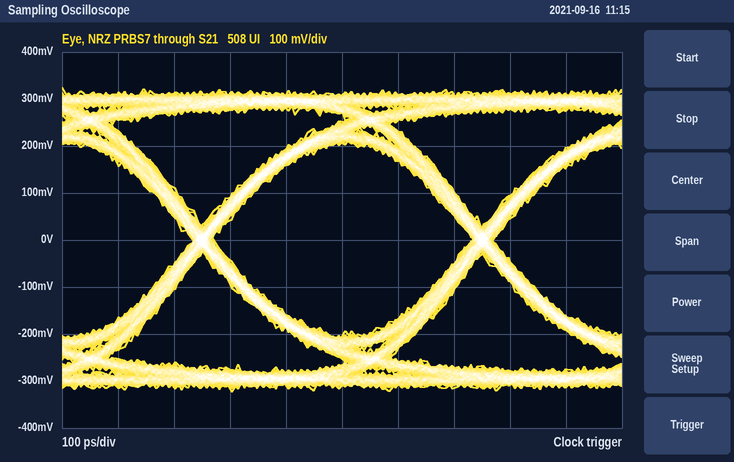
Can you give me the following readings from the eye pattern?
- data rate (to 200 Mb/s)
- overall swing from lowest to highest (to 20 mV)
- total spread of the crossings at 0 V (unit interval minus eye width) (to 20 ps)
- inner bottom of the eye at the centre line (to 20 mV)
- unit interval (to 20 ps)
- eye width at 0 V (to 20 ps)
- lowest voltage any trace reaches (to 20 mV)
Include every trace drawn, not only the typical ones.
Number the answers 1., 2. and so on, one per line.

1. 2.0 Gb/s
2. 640 mV
3. 40 ps
4. -200 mV
5. 500 ps
6. 460 ps
7. -320 mV
